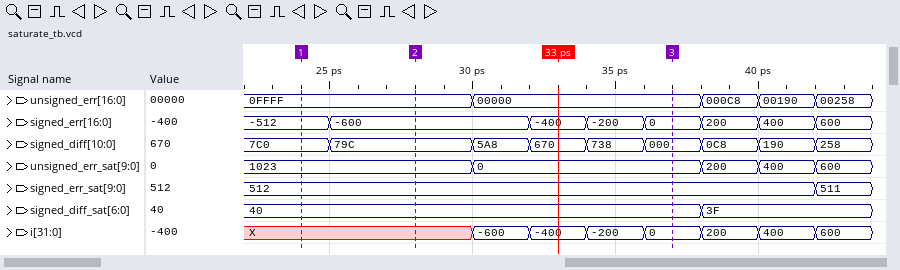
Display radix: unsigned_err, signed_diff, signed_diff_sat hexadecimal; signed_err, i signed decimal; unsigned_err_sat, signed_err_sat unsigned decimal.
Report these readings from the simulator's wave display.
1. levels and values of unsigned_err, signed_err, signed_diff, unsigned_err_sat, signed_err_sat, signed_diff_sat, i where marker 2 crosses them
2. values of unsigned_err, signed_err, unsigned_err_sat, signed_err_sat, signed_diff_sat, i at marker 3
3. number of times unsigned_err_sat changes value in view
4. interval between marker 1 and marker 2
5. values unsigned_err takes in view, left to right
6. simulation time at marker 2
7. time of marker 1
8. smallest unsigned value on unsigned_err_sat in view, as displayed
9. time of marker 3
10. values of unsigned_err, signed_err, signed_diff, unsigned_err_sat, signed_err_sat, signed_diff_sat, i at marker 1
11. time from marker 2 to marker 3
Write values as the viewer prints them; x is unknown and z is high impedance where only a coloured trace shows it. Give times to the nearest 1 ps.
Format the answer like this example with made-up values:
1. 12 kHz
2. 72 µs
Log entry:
1. unsigned_err=0FFFF, signed_err=-600, signed_diff=79C, unsigned_err_sat=1023, signed_err_sat=512, signed_diff_sat=40, i=X
2. unsigned_err=00000, signed_err=0, unsigned_err_sat=0, signed_err_sat=512, signed_diff_sat=40, i=0
3. 4
4. 4 ps
5. 0FFFF, 00000, 000C8, 00190, 00258
6. 28 ps
7. 24 ps
8. 0
9. 37 ps
10. unsigned_err=0FFFF, signed_err=-512, signed_diff=7C0, unsigned_err_sat=1023, signed_err_sat=512, signed_diff_sat=40, i=X
11. 9 ps
